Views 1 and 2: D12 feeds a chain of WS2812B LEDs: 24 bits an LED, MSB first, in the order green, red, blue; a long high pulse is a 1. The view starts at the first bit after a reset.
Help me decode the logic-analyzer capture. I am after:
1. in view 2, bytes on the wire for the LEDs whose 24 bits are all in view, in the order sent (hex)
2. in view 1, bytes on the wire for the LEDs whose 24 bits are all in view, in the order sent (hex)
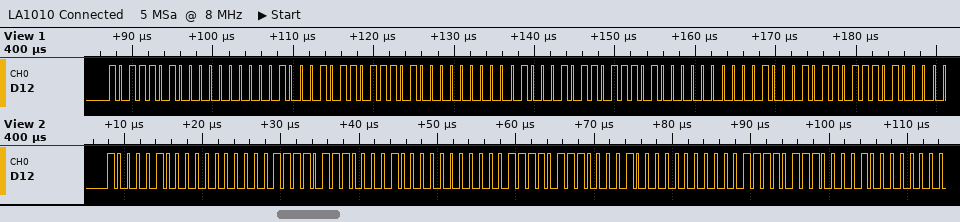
84 00 7B 84 00 7B 84 00 7B
BA 00 45 BA 00 45 BA 00 45
